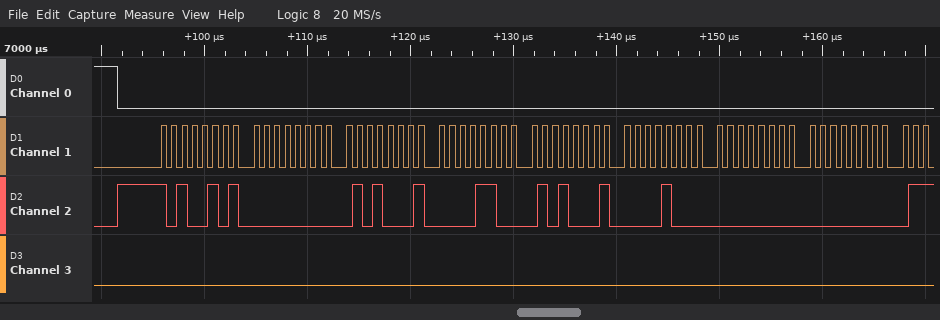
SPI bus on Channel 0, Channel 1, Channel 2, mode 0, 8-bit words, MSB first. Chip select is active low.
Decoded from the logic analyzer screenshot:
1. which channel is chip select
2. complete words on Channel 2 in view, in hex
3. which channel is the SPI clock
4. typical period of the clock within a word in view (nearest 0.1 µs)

Channel 0
A5, 00, 51, 0C, 51, 08, 00, 00
Channel 1
1 µs
